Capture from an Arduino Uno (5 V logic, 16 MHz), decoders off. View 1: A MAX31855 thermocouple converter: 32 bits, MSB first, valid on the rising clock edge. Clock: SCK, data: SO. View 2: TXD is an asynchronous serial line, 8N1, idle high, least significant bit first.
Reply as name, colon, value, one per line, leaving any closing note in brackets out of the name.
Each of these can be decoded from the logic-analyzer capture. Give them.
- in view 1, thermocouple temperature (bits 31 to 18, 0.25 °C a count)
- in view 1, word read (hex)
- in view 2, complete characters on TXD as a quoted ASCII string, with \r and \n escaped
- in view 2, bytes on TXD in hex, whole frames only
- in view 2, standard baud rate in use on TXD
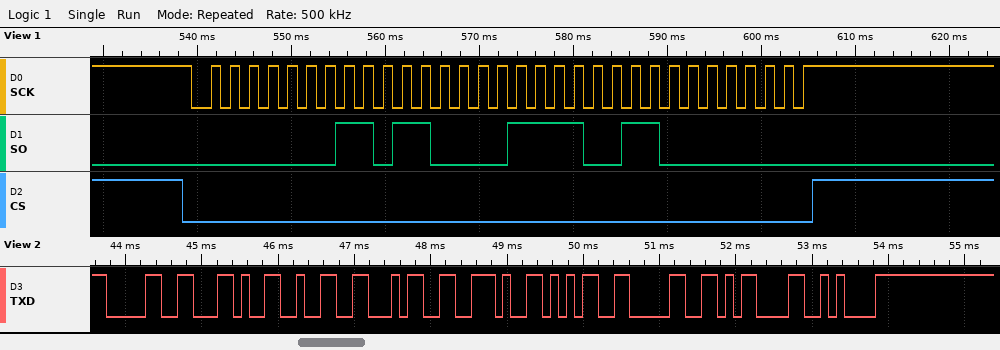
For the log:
in view 1, thermocouple temperature: 27.00 °C
in view 1, word read: 0x01B0F300
in view 2, complete characters on TXD as a quoted ASCII string, with \r and \n escaped: "0,24.50\r\n"
in view 2, bytes on TXD in hex, whole frames only: 0x30 0x2C 0x32 0x34 0x2E 0x35 0x30 0x0D 0x0A
in view 2, standard baud rate in use on TXD: 9600 baud
